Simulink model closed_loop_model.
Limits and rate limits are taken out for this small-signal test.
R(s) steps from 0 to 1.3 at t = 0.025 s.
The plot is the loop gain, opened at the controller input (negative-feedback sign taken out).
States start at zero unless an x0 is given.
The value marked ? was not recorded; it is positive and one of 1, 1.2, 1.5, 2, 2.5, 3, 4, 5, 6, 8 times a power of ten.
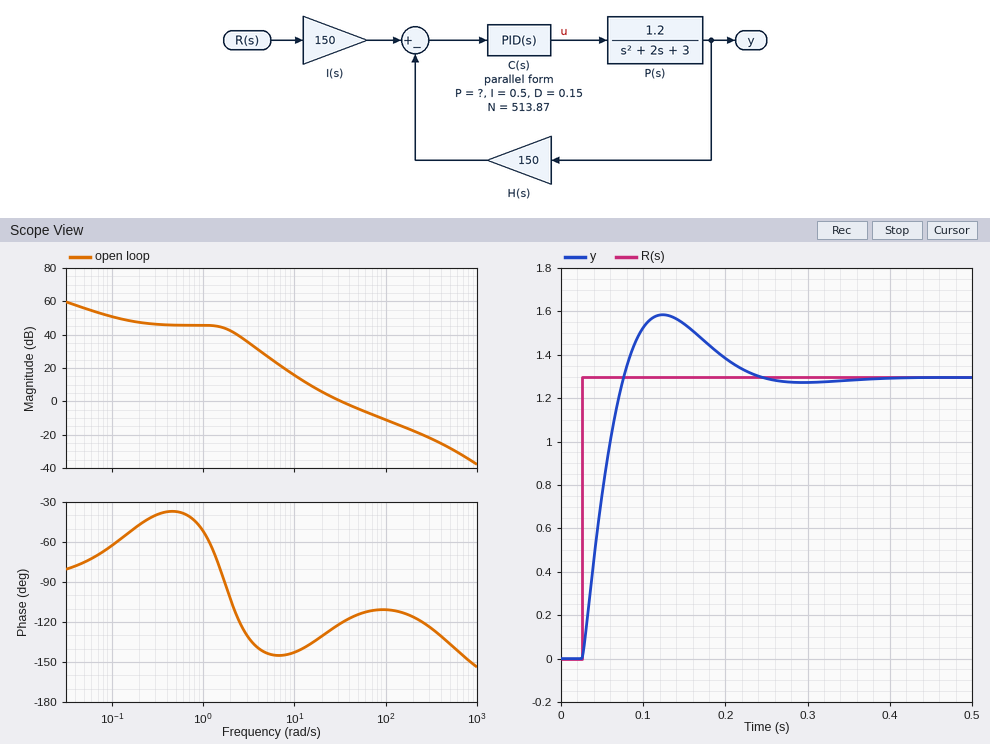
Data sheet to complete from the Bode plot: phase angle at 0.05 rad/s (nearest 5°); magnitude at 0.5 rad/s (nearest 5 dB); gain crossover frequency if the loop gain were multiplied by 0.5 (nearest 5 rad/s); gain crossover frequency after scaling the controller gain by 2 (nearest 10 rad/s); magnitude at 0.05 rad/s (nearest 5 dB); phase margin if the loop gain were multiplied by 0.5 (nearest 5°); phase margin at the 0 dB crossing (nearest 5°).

-75°
45 dB
20 rad/s
60 rad/s
55 dB
50°
60°
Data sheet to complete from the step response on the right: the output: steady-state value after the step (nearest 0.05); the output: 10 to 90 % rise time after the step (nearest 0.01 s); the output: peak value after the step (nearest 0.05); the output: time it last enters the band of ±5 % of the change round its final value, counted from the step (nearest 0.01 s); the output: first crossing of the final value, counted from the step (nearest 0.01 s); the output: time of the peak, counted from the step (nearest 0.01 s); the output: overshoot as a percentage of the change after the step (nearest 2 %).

1.30
0.04 s
1.60
0.18 s
0.05 s
0.10 s
22 %
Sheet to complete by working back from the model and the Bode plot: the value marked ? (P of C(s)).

3
